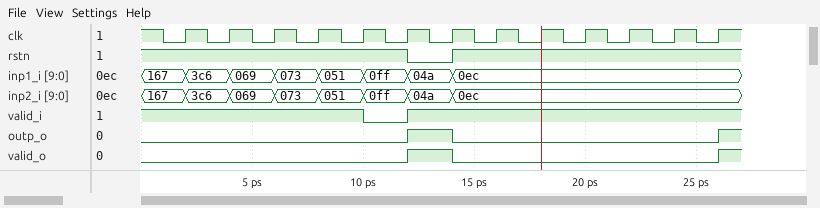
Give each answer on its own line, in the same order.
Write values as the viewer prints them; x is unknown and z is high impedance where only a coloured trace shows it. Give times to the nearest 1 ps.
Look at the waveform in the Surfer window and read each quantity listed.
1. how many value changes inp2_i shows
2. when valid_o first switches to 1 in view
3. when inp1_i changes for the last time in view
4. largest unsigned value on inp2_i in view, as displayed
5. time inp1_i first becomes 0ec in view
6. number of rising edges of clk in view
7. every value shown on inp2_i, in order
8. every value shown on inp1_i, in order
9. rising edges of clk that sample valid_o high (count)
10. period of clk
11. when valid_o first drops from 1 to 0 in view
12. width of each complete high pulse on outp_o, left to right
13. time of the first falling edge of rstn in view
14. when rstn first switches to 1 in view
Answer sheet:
7
12 ps
14 ps
3c6
14 ps
13
167, 3c6, 069, 073, 051, 0ff, 04a, 0ec
167, 3c6, 069, 073, 051, 0ff, 04a, 0ec
1
2 ps
14 ps
2 ps
12 ps
14 ps
